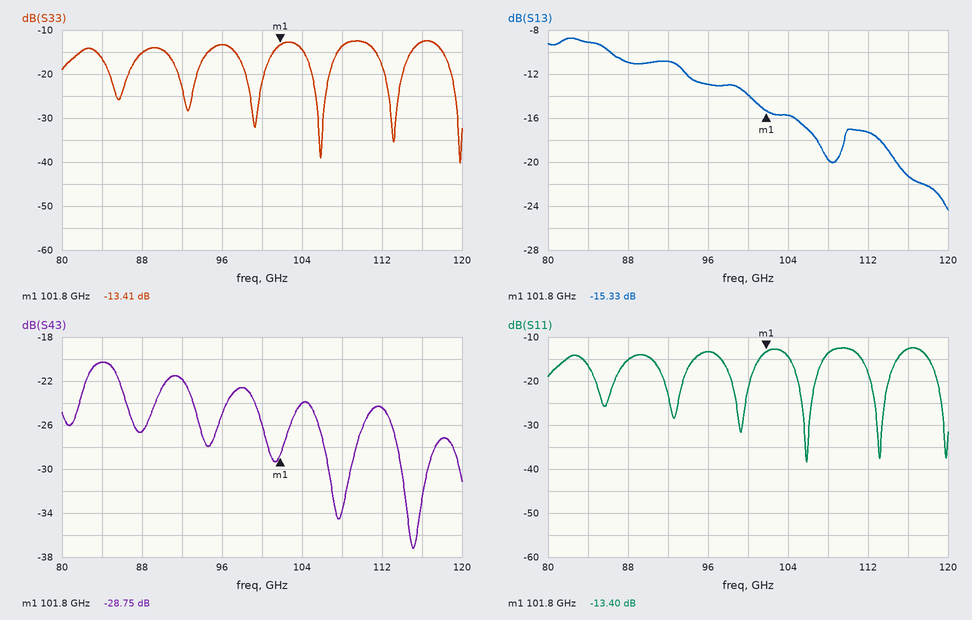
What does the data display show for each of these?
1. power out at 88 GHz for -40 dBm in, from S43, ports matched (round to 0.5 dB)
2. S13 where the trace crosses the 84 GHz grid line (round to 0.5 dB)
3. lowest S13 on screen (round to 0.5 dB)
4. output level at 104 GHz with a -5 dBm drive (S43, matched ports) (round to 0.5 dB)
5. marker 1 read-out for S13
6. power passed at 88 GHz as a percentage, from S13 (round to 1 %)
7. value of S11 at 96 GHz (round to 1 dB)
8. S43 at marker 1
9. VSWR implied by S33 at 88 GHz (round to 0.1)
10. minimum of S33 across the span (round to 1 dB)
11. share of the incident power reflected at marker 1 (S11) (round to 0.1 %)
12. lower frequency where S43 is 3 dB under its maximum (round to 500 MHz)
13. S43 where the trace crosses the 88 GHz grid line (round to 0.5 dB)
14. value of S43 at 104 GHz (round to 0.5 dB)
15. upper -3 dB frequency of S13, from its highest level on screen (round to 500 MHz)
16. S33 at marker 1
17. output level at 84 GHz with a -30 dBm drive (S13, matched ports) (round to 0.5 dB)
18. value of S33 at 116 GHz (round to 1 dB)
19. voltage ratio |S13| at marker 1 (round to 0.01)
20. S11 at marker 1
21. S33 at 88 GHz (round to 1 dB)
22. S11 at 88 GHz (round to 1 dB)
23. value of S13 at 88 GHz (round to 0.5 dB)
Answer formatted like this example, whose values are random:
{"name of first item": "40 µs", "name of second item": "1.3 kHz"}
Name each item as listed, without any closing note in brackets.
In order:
{"power out at 88 GHz for -40 dBm in, from S43, ports matched": "-66.5 dBm", "S13 where the trace crosses the 84 GHz grid line": "-9.0 dB", "lowest S13 on screen": "-24.5 dB", "output level at 104 GHz with a -5 dBm drive (S43, matched ports)": "-29.0 dBm", "marker 1 read-out for S13": "-15.33 dB", "power passed at 88 GHz as a percentage, from S13": "8 %", "value of S11 at 96 GHz": "-13 dB", "S43 at marker 1": "-28.75 dB", "VSWR implied by S33 at 88 GHz": "1.4", "minimum of S33 across the span": "-40 dB", "share of the incident power reflected at marker 1 (S11)": "4.6 %", "lower frequency where S43 is 3 dB under its maximum": "82.0 GHz", "S43 where the trace crosses the 88 GHz grid line": "-26.5 dB", "value of S43 at 104 GHz": "-24.0 dB", "upper -3 dB frequency of S13, from its highest level on screen": "93.5 GHz", "S33 at marker 1": "-13.41 dB", "output level at 84 GHz with a -30 dBm drive (S13, matched ports)": "-39.0 dBm", "value of S33 at 116 GHz": "-13 dB", "voltage ratio |S13| at marker 1": "0.17", "S11 at marker 1": "-13.40 dB", "S33 at 88 GHz": "-15 dB", "S11 at 88 GHz": "-15 dB", "value of S13 at 88 GHz": "-11.0 dB"}
